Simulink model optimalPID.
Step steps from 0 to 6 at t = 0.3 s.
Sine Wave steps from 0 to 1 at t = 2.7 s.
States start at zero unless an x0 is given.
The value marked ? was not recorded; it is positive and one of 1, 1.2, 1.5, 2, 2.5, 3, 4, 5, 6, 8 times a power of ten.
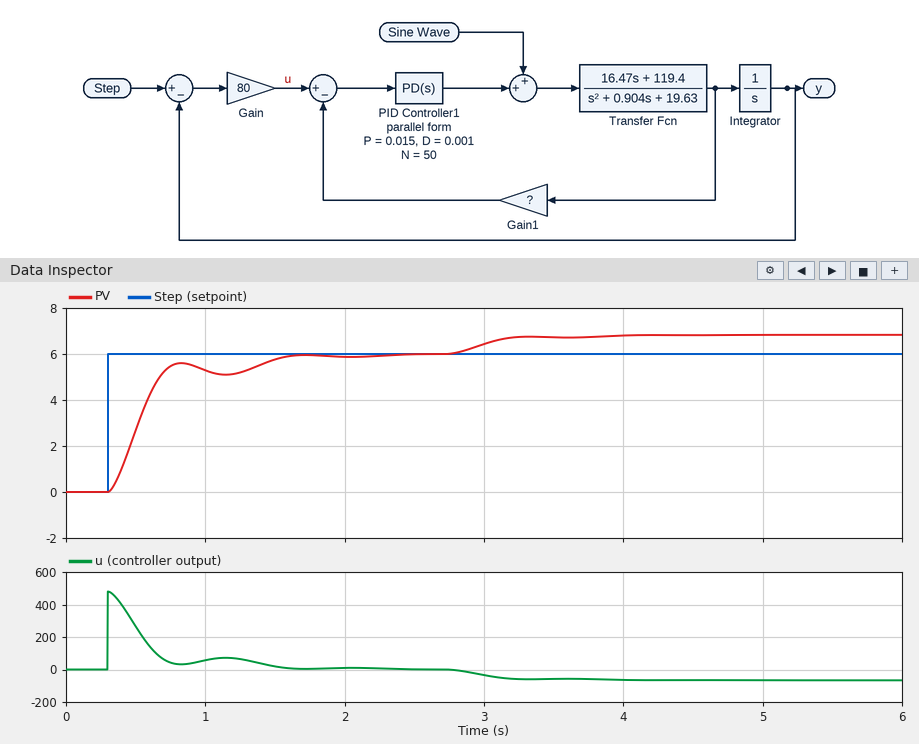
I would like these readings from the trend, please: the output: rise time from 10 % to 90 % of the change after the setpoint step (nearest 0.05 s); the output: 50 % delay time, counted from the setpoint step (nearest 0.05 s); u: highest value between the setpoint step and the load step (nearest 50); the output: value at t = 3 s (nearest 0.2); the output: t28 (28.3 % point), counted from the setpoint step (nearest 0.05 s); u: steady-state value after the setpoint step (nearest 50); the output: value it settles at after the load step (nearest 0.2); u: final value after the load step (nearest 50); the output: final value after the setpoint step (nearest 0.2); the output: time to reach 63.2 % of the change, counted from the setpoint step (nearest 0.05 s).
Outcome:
0.35 s
0.20 s
500
6.4
0.15 s
0
6.8
-50
6.0
0.25 s
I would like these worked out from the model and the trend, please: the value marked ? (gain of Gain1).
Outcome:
15
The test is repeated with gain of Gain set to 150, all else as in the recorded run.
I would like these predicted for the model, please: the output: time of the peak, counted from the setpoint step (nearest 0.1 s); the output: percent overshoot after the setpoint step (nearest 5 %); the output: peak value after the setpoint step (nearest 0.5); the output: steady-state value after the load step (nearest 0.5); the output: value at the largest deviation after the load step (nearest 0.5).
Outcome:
0.4 s
10 %
6.5
6.5
6.5
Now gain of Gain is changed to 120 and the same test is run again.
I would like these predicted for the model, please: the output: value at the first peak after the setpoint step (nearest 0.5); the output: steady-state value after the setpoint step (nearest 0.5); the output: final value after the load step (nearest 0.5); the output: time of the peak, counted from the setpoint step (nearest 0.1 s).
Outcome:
6.5
6.0
6.5
0.4 s
